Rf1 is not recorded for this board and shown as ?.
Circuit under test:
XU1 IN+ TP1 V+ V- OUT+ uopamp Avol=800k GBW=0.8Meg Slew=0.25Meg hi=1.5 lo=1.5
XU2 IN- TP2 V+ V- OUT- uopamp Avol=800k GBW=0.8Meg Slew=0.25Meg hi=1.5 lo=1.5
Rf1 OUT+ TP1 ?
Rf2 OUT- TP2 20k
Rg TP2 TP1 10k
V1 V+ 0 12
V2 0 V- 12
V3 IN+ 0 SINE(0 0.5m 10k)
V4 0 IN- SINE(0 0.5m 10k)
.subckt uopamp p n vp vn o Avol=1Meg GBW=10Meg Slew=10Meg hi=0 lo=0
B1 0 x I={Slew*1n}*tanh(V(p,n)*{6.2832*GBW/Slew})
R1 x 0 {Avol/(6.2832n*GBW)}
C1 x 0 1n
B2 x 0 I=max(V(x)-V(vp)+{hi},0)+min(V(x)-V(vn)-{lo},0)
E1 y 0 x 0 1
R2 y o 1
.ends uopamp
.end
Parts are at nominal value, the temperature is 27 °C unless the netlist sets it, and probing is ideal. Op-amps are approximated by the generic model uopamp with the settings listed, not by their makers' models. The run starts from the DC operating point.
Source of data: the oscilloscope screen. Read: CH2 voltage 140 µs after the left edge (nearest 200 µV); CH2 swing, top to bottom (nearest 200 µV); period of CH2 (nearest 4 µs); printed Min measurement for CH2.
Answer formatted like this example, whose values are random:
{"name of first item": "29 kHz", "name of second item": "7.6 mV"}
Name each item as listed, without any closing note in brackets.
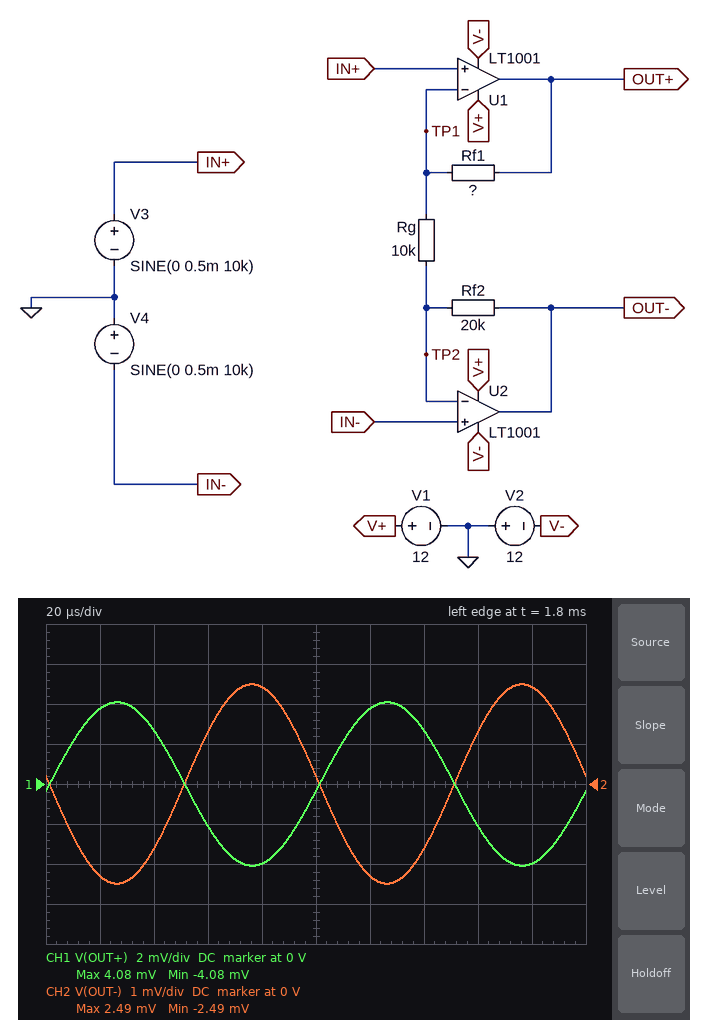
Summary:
{"CH2 voltage 140 µs after the left edge": "-1.6 mV", "CH2 swing, top to bottom": "5.0 mV", "period of CH2": "100 µs", "printed Min measurement for CH2": "-2.49 mV"}
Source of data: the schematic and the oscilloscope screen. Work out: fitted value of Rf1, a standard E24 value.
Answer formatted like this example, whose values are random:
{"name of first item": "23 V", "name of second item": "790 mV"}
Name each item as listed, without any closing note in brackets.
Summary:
{"fitted value of Rf1, a standard E24 value": "36 kΩ"}
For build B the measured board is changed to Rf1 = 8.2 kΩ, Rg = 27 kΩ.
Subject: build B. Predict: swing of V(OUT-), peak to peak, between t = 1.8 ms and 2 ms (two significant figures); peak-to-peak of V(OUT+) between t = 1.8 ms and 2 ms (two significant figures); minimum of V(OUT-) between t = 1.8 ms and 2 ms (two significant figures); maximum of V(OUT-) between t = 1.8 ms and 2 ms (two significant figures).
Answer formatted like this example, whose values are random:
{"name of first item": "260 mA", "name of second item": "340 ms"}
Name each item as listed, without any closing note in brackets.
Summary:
{"swing of V(OUT-), peak to peak, between t = 1.8 ms and 2 ms": "2.5 mV", "peak-to-peak of V(OUT+) between t = 1.8 ms and 2 ms": "1.6 mV", "minimum of V(OUT-) between t = 1.8 ms and 2 ms": "-1.2 mV", "maximum of V(OUT-) between t = 1.8 ms and 2 ms": "1.2 mV"}
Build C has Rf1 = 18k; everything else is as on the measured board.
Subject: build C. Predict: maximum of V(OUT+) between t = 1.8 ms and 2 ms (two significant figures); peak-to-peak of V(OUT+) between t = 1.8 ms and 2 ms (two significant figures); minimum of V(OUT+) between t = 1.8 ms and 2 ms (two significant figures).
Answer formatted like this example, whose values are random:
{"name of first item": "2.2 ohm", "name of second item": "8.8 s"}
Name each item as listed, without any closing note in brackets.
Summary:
{"maximum of V(OUT+) between t = 1.8 ms and 2 ms": "2.3 mV", "peak-to-peak of V(OUT+) between t = 1.8 ms and 2 ms": "4.6 mV", "minimum of V(OUT+) between t = 1.8 ms and 2 ms": "-2.3 mV"}
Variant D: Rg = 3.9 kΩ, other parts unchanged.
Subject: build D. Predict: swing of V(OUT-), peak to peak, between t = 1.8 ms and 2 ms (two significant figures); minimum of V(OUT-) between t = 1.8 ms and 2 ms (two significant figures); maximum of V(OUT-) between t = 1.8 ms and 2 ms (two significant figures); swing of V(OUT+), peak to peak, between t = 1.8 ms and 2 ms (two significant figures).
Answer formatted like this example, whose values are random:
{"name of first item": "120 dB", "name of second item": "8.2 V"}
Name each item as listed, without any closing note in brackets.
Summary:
{"swing of V(OUT-), peak to peak, between t = 1.8 ms and 2 ms": "11 mV", "minimum of V(OUT-) between t = 1.8 ms and 2 ms": "-5.5 mV", "maximum of V(OUT-) between t = 1.8 ms and 2 ms": "5.5 mV", "swing of V(OUT+), peak to peak, between t = 1.8 ms and 2 ms": "19 mV"}
